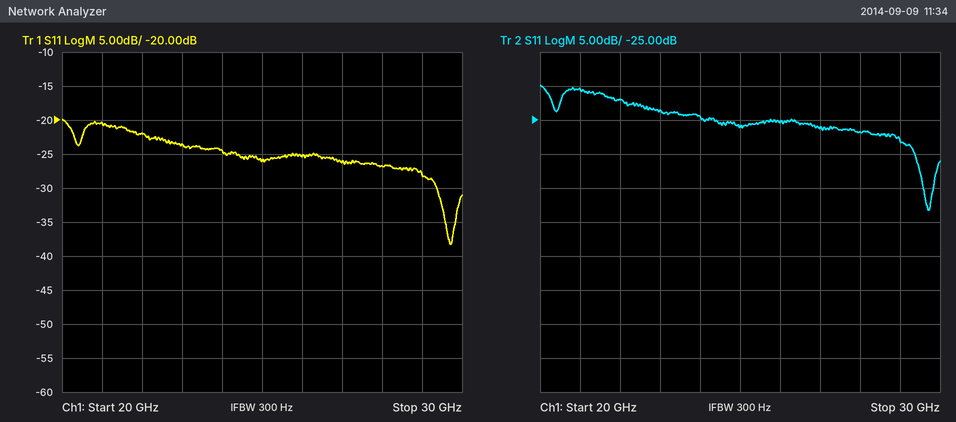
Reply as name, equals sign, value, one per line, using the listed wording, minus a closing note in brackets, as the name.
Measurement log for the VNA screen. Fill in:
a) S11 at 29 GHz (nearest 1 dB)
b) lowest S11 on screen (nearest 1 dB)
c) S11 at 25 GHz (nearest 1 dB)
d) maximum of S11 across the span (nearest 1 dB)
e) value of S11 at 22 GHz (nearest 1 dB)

S11 at 29 GHz = -28 dB
lowest S11 on screen = -38 dB
S11 at 25 GHz = -26 dB
maximum of S11 across the span = -20 dB
value of S11 at 22 GHz = -22 dB
